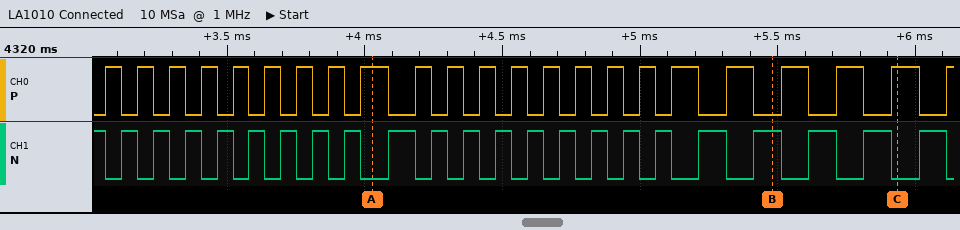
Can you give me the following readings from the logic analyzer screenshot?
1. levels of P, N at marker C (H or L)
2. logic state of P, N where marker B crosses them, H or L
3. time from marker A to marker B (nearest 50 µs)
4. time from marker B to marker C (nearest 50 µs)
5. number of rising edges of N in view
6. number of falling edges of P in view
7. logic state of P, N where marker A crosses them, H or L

P=H, N=L
P=L, N=H
1450 µs
450 µs
22
22
P=H, N=L
